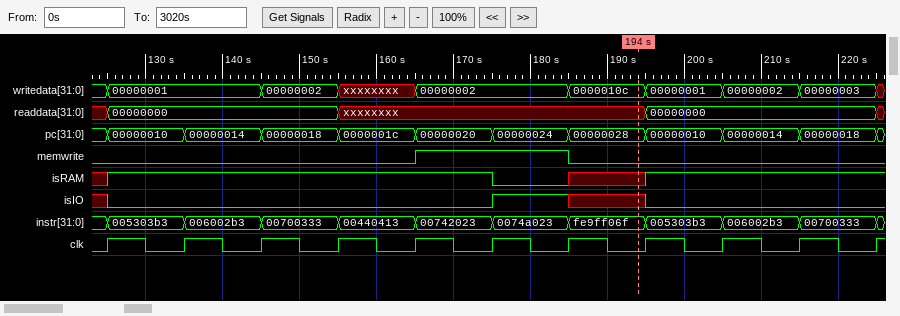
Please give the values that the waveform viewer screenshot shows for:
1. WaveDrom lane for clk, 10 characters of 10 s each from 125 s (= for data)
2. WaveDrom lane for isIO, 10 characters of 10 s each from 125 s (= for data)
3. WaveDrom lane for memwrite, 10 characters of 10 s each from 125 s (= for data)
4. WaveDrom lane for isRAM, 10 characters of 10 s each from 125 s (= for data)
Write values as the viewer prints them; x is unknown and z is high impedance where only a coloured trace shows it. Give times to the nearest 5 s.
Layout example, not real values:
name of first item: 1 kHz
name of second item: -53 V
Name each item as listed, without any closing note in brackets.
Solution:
WaveDrom lane for clk, 10 characters of 10 s each from 125 s: {name: 'clk', wave: 'p.........'}
WaveDrom lane for isIO, 10 characters of 10 s each from 125 s: {name: 'isIO', wave: '0....1x0..'}
WaveDrom lane for memwrite, 10 characters of 10 s each from 125 s: {name: 'memwrite', wave: '0...1.0...'}
WaveDrom lane for isRAM, 10 characters of 10 s each from 125 s: {name: 'isRAM', wave: '1....0x1..'}
